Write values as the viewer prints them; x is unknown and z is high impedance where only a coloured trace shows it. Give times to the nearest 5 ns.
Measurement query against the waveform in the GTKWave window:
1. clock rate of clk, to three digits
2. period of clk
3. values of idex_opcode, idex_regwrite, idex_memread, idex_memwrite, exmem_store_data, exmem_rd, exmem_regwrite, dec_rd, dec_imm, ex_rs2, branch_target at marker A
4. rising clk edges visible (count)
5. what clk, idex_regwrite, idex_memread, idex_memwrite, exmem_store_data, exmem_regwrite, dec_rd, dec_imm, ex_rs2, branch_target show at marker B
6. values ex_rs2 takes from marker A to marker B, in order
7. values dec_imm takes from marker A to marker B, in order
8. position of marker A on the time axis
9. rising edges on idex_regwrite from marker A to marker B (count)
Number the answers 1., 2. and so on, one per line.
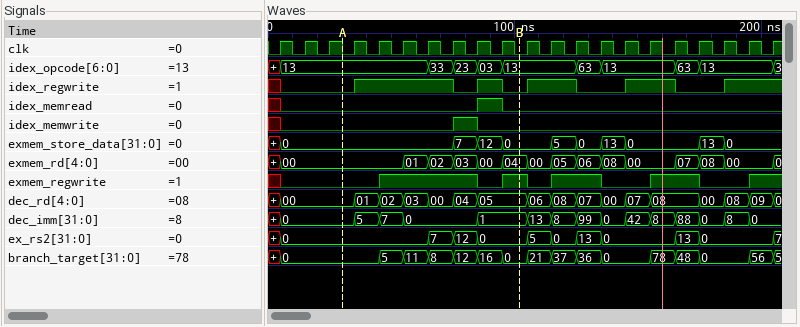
1. 100 MHz
2. 10 ns
3. idex_opcode=13, idex_regwrite=0, idex_memread=0, idex_memwrite=0, exmem_store_data=0, exmem_rd=00, exmem_regwrite=0, dec_rd=00, dec_imm=0, ex_rs2=0, branch_target=0
4. 21
5. clk=0, idex_regwrite=0, idex_memread=0, idex_memwrite=0, exmem_store_data=0, exmem_regwrite=1, dec_rd=05, dec_imm=1, ex_rs2=0, branch_target=0
6. 0, 7, 12, 0
7. 0, 5, 7, 0, 1
8. 30 ns
9. 2
